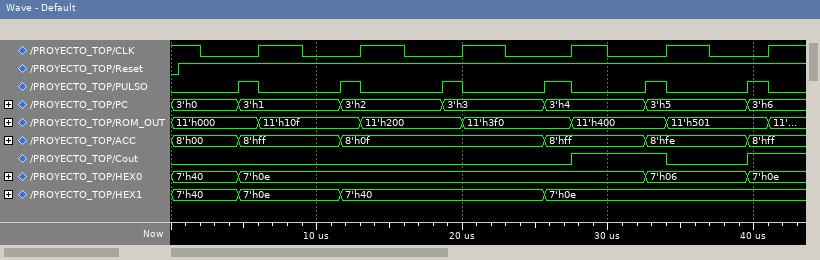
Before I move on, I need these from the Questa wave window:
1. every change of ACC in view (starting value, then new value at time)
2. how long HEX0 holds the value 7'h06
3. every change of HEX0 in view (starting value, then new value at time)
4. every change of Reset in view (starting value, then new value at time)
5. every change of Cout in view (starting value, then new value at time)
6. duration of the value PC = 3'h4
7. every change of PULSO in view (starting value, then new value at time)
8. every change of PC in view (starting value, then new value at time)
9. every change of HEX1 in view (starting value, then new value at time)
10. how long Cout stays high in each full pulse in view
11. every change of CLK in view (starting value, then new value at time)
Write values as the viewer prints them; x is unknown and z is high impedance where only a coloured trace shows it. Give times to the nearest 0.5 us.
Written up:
8'h00, 8'hff at 4.5 us, 8'h0f at 11.5 us, 8'hff at 25.5 us, 8'hfe at 32.5 us, 8'hff at 39.5 us
7 us
7'h40, 7'h0e at 4.5 us, 7'h06 at 32.5 us, 7'h0e at 39.5 us
0, 1 at 0.5 us
0, 1 at 27.5 us, 0 at 34 us, 1 at 39.5 us
7 us
0, 1 at 4.5 us, 0 at 6 us, 1 at 11.5 us, 0 at 13 us, 1 at 18.5 us, 0 at 20 us, 1 at 25.5 us, 0 at 27.5 us, 1 at 32.5 us, 0 at 34 us, 1 at 39.5 us, 0 at 41 us
3'h0, 3'h1 at 4.5 us, 3'h2 at 11.5 us, 3'h3 at 18.5 us, 3'h4 at 25.5 us, 3'h5 at 32.5 us, 3'h6 at 39.5 us
7'h40, 7'h0e at 4.5 us, 7'h40 at 11.5 us, 7'h0e at 25.5 us
6.5 us
1, 0 at 2 us, 1 at 6 us, 0 at 9 us, 1 at 13 us, 0 at 16 us, 1 at 20 us, 0 at 23 us, 1 at 27.5 us, 0 at 30 us, 1 at 34 us, 0 at 37 us, 1 at 41 us
